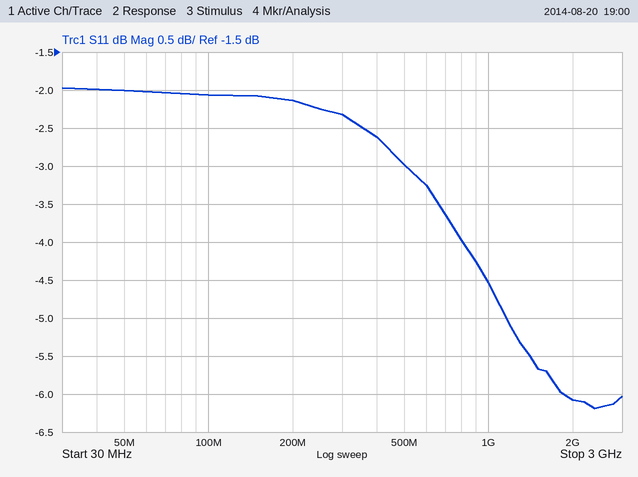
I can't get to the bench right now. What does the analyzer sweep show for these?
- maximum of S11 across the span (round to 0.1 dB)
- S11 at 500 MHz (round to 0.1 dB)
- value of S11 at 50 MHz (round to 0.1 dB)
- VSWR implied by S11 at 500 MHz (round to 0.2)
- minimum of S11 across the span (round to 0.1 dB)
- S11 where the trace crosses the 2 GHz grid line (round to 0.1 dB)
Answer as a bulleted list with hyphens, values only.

- -2.0 dB
- -3.0 dB
- -2.0 dB
- 5.8
- -6.2 dB
- -6.1 dB
